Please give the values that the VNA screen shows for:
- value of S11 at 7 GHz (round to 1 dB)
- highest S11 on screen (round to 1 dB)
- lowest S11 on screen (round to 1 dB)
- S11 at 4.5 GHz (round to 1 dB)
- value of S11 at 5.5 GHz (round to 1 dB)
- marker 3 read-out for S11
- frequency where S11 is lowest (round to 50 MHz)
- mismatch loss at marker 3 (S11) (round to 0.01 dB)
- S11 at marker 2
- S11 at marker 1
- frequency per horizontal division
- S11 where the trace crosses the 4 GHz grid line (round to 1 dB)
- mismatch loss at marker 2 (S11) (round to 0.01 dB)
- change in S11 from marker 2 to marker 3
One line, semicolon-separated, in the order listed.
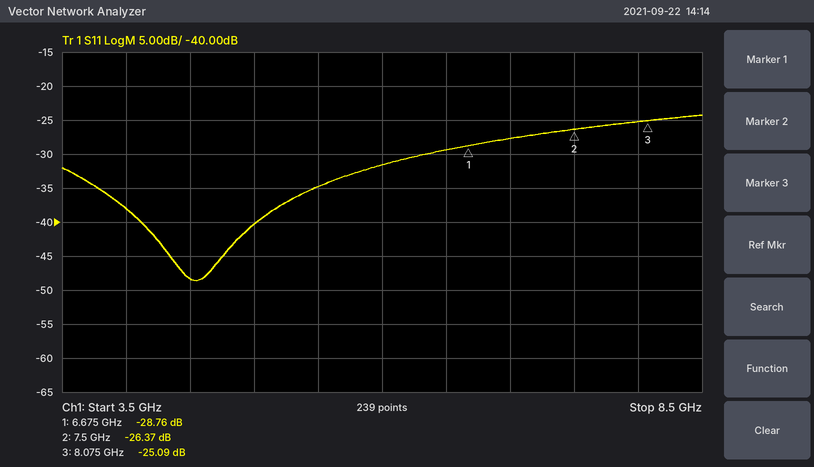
-28 dB; -24 dB; -49 dB; -48 dB; -35 dB; -25.09 dB; 4.55 GHz; 0.01 dB; -26.37 dB; -28.76 dB; 500 MHz; -38 dB; 0.01 dB; 1.28 dB
